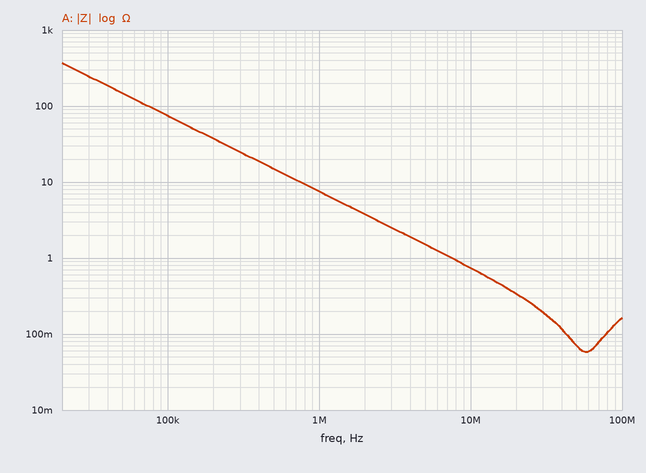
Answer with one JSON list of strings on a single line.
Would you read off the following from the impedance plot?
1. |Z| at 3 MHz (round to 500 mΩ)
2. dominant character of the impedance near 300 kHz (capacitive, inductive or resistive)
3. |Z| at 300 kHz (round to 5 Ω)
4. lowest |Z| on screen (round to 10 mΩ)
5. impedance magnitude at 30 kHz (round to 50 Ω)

["2.5 Ω", "capacitive", "25 Ω", "60 mΩ", "250 Ω"]
